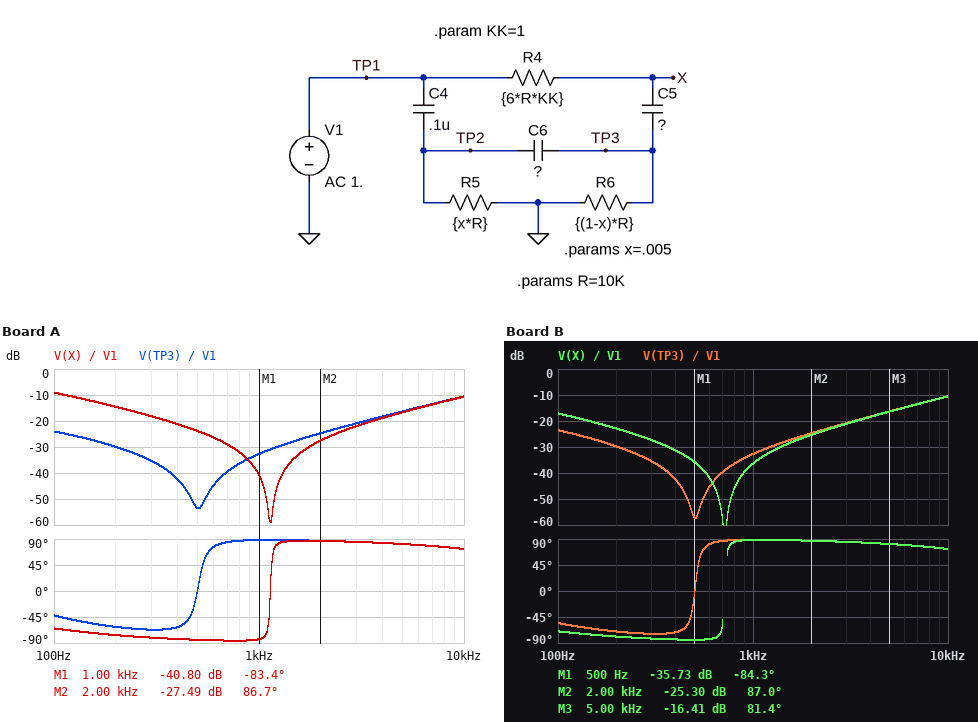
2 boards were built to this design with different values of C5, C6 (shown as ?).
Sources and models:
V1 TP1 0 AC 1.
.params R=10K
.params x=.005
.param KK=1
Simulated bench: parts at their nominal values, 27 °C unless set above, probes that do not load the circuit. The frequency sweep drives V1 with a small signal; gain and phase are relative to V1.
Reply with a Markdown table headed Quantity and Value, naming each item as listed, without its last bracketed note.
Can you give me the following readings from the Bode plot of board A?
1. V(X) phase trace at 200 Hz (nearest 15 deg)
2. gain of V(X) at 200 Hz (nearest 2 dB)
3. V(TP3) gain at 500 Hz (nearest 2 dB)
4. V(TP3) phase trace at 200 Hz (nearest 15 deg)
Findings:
| Quantity | Value |
|---|---|
| V(X) phase trace at 200 Hz | -75 deg |
| gain of V(X) at 200 Hz | -14 dB |
| V(TP3) gain at 500 Hz | -54 dB |
| V(TP3) phase trace at 200 Hz | -60 deg |
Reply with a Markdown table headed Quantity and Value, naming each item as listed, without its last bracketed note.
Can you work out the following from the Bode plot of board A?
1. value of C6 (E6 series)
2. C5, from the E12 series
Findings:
| Quantity | Value |
|---|---|
| value of C6 | 330 nF |
| C5, from the E12 series | 82 nF |
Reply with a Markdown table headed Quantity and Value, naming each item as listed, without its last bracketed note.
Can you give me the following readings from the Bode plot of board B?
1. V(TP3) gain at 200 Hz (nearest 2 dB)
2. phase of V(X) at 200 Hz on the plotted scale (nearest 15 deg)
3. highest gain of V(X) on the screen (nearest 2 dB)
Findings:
| Quantity | Value |
|---|---|
| V(TP3) gain at 200 Hz | -30 dB |
| phase of V(X) at 200 Hz on the plotted scale | -75 deg |
| highest gain of V(X) on the screen | -10 dB |
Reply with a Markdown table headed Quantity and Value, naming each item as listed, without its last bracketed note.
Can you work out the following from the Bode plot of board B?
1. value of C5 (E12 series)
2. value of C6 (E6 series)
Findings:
| Quantity | Value |
|---|---|
| value of C5 | 330 nF |
| value of C6 | 330 nF |
